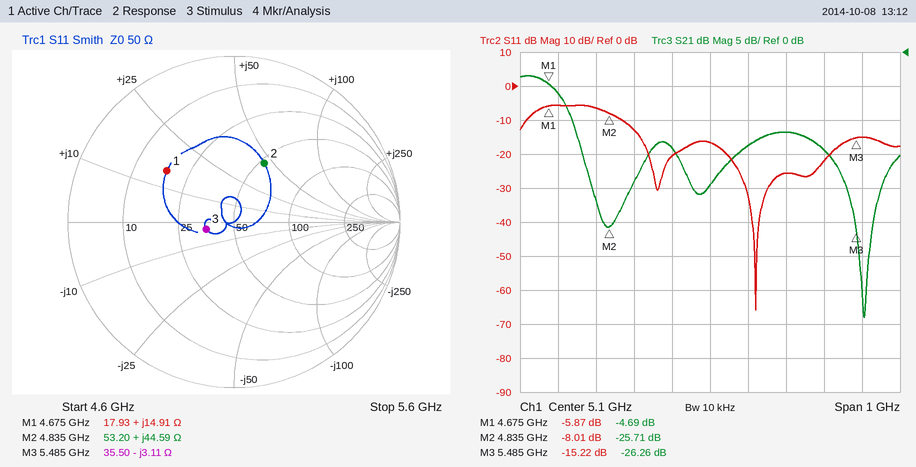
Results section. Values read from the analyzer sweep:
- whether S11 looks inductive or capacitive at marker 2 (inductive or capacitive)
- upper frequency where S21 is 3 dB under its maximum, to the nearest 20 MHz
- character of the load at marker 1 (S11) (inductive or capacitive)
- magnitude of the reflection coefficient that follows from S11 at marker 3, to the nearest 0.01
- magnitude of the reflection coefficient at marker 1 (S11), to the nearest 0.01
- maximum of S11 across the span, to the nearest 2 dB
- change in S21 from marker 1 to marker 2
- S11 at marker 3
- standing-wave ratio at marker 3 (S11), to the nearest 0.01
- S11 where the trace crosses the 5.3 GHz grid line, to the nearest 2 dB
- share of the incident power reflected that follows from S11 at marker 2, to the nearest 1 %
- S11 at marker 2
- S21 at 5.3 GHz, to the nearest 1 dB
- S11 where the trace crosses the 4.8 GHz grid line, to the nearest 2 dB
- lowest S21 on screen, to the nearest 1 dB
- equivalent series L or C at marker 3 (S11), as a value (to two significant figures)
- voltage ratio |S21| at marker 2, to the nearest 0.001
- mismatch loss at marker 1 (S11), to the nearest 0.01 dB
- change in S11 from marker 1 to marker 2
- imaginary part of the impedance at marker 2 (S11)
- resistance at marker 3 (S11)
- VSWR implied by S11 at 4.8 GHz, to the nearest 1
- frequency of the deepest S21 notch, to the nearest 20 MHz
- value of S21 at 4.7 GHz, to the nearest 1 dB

inductive
4.70 GHz
inductive
0.17
0.51
-6 dB
-21.02 dB
-15.22 dB
1.42
-26 dB
16 %
-8.01 dB
-12 dB
-6 dB
-39 dB
9.3 pF
0.052
1.30 dB
-2.14 dB
+44.59 Ω
35.50 Ω
3
5.50 GHz
-6 dB
